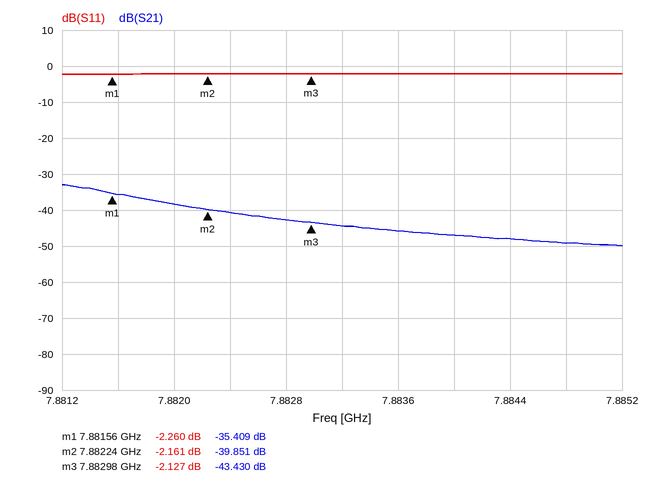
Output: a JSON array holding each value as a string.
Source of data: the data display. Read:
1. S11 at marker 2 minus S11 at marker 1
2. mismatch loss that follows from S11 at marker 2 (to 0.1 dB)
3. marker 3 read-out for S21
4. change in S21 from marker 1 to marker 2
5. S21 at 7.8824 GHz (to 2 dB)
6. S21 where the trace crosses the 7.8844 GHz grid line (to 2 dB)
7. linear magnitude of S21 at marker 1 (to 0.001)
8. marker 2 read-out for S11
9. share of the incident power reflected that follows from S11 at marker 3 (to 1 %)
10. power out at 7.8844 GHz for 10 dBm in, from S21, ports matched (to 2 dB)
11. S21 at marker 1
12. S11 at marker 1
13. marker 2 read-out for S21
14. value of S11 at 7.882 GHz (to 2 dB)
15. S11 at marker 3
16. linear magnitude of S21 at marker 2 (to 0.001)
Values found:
["0.099 dB", "4.1 dB", "-43.430 dB", "-4.442 dB", "-40 dB", "-48 dB", "0.017", "-2.161 dB", "61 %", "-38 dBm", "-35.409 dB", "-2.260 dB", "-39.851 dB", "-2 dB", "-2.127 dB", "0.010"]
